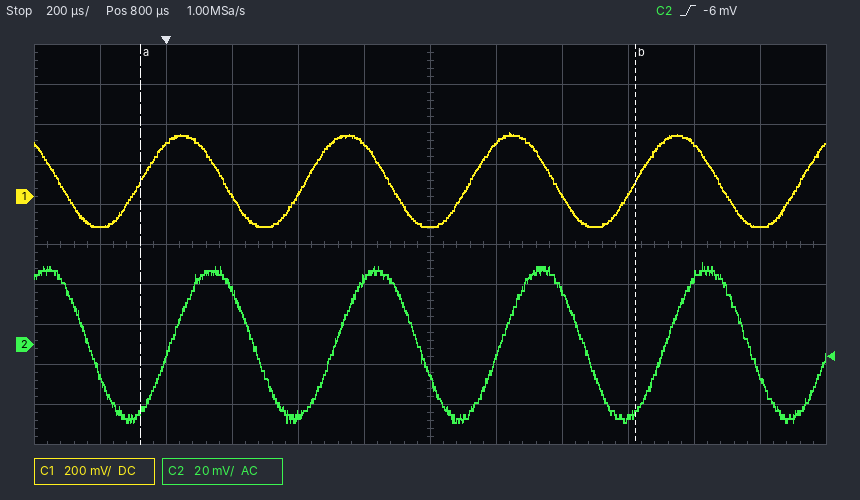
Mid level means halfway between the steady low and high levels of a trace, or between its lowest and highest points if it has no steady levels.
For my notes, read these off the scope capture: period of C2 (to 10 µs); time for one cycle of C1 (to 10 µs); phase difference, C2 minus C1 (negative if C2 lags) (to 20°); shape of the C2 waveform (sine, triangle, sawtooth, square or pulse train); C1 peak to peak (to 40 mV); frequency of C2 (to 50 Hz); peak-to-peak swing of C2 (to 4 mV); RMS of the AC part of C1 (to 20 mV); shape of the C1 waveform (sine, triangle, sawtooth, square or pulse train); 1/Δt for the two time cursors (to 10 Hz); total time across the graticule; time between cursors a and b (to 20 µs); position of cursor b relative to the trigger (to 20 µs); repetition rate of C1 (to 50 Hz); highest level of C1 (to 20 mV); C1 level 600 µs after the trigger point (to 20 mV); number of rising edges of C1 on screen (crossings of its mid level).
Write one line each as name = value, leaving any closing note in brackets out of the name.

period of C2 = 500 µs
time for one cycle of C1 = 500 µs
phase difference, C2 minus C1 (negative if C2 lags) = -60°
shape of the C2 waveform = sine
C1 peak to peak = 480 mV
frequency of C2 = 2.00 kHz
peak-to-peak swing of C2 = 80 mV
RMS of the AC part of C1 = 160 mV
shape of the C1 waveform = sine
1/Δt for the two time cursors = 670 Hz
total time across the graticule = 2.4 ms
time between cursors a and b = 1.50 ms
position of cursor b relative to the trigger = +1.42 ms
repetition rate of C1 = 2.00 kHz
highest level of C1 = 320 mV
C1 level 600 µs after the trigger point = 260 mV
number of rising edges of C1 on screen = 5
